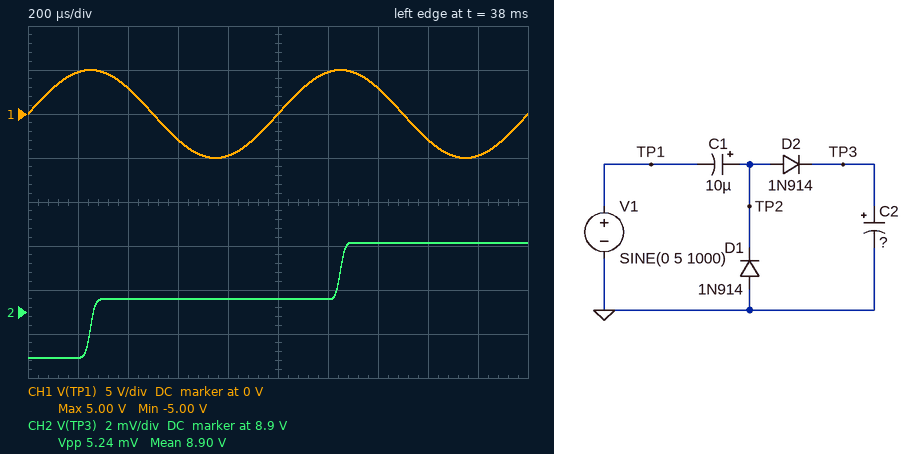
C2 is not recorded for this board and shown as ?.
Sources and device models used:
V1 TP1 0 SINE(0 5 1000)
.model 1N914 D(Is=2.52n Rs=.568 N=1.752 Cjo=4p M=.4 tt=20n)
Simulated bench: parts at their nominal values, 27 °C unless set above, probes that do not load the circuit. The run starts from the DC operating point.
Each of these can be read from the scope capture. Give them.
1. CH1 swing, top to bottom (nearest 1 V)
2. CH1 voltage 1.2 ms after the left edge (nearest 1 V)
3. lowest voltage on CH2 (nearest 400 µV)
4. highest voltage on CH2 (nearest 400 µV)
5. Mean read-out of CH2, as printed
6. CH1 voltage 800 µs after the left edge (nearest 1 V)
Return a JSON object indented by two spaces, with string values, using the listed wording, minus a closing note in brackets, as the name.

{
  "CH1 swing, top to bottom": "10 V",
  "CH1 voltage 1.2 ms after the left edge": "5 V",
  "lowest voltage on CH2": "8.8980 V",
  "highest voltage on CH2": "8.9032 V",
  "Mean read-out of CH2, as printed": "8.90 V",
  "CH1 voltage 800 µs after the left edge": "-5 V"
}
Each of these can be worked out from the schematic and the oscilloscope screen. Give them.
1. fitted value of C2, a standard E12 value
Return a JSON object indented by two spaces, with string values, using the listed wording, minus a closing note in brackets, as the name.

{
  "fitted value of C2, a standard E12 value": "4.7 µF"
}
